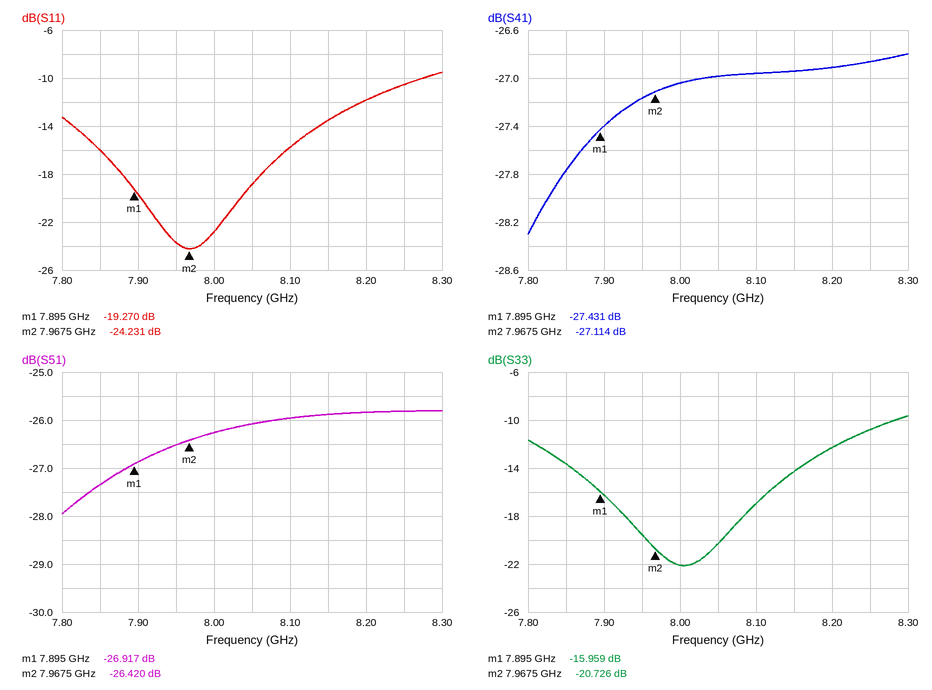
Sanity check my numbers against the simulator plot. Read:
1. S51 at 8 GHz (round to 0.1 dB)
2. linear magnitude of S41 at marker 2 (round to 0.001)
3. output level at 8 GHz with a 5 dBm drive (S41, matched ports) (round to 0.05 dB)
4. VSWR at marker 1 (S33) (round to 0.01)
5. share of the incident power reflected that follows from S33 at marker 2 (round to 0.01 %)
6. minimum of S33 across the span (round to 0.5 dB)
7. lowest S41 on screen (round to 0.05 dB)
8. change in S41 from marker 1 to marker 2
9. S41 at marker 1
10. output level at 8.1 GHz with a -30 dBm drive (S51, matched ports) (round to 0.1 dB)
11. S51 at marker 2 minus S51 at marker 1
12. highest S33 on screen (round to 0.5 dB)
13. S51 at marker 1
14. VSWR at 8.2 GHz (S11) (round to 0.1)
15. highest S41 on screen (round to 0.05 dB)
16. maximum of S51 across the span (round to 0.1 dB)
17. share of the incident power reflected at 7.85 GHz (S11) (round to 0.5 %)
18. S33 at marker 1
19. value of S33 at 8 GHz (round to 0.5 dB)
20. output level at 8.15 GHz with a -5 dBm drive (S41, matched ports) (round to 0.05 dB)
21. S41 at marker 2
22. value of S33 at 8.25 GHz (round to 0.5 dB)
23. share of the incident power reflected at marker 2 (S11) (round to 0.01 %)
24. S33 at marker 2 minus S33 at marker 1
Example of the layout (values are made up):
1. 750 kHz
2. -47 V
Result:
1. -26.3 dB
2. 0.044
3. -22.05 dBm
4. 1.38
5. 0.85 %
6. -22.0 dB
7. -28.30 dB
8. 0.317 dB
9. -27.431 dB
10. -56.0 dBm
11. 0.497 dB
12. -9.5 dB
13. -26.917 dB
14. 1.7
15. -26.80 dB
16. -25.8 dB
17. 2.5 %
18. -15.959 dB
19. -22.0 dB
20. -31.95 dBm
21. -27.114 dB
22. -11.0 dB
23. 0.38 %
24. -4.767 dB
